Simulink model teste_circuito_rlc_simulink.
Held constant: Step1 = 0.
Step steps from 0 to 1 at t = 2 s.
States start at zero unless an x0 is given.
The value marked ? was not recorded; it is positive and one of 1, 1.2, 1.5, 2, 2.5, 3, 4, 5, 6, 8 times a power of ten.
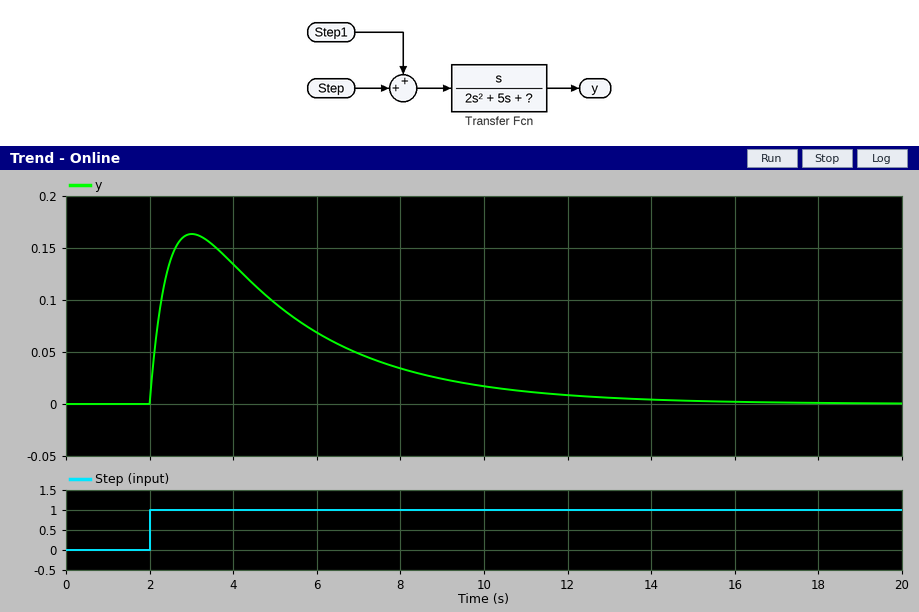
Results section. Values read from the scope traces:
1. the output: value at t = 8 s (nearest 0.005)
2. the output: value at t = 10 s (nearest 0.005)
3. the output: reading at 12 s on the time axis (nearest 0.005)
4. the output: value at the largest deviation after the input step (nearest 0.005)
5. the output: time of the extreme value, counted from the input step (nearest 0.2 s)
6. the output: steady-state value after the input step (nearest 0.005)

0.035
0.015
0.010
0.165
1.0 s
0.000
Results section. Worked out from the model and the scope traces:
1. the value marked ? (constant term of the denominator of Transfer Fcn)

1.5
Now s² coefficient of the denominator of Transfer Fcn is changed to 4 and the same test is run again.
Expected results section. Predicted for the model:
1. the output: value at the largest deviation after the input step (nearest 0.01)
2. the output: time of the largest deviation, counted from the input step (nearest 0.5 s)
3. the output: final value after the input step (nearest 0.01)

0.15
1.5 s
0.00
